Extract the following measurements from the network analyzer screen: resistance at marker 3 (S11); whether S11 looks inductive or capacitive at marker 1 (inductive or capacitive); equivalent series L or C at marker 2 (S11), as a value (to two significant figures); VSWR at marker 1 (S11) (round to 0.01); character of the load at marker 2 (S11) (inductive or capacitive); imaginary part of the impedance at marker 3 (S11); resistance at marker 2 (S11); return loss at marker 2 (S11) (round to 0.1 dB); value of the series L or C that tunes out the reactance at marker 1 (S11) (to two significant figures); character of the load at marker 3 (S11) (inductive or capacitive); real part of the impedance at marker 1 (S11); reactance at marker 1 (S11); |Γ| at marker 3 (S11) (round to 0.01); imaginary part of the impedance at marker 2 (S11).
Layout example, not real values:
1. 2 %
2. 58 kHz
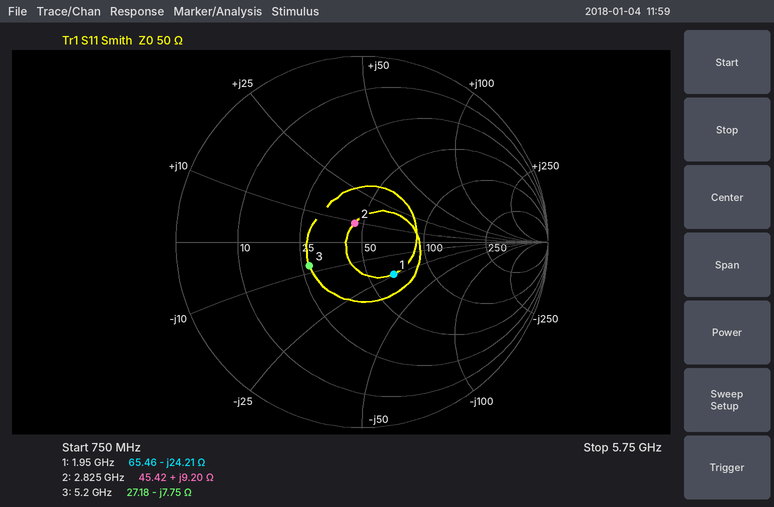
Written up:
1. 27.18 Ω
2. capacitive
3. 520 pH
4. 1.64
5. inductive
6. -7.75 Ω
7. 45.42 Ω
8. 19.4 dB
9. 2.0 nH
10. capacitive
11. 65.46 Ω
12. -24.21 Ω
13. 0.31
14. +9.20 Ω
